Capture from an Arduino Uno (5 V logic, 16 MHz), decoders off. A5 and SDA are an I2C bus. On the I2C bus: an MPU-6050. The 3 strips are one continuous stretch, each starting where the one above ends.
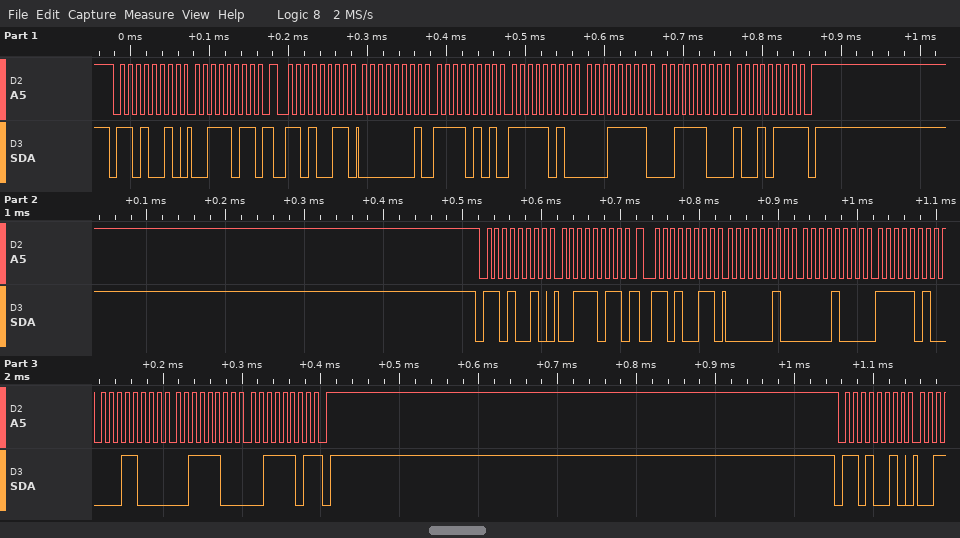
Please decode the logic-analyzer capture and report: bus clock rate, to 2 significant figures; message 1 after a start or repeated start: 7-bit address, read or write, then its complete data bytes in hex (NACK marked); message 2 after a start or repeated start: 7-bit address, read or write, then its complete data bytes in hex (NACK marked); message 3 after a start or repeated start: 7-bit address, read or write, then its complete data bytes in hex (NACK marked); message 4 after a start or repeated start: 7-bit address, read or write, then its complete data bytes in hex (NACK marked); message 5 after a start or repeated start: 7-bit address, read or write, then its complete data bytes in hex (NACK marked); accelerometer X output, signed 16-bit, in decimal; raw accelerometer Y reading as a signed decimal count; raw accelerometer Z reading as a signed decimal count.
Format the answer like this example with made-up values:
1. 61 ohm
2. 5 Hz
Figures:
1. 100 kHz
2. 0x69 write: 3B
3. 0x69 read: 01 F5 FA 1F 3C 97 NACK
4. 0x69 write: 3B
5. 0x69 read: 02 08 FA 18 3C 3D NACK
6. 0x69 write
7. 501
8. -1505
9. 15511
